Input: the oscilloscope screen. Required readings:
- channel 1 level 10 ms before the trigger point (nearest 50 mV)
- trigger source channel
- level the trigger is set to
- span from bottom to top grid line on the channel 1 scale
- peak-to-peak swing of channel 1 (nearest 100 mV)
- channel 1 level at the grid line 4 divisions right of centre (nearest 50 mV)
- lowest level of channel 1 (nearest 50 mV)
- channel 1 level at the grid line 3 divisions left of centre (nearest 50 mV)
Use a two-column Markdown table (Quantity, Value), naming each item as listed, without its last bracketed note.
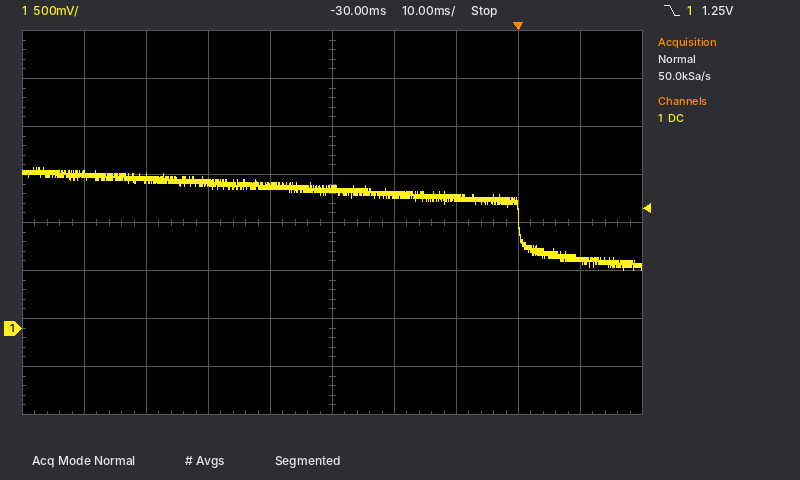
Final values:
| Quantity | Value |
|---|---|
| channel 1 level 10 ms before the trigger point | 1.35 V |
| trigger source channel | channel 1 |
| level the trigger is set to | 1.25 V |
| span from bottom to top grid line on the channel 1 scale | 4 V |
| peak-to-peak swing of channel 1 | 1.10 V |
| channel 1 level at the grid line 4 divisions right of centre | 700 mV |
| lowest level of channel 1 | 600 mV |
| channel 1 level at the grid line 3 divisions left of centre | 1.55 V |
